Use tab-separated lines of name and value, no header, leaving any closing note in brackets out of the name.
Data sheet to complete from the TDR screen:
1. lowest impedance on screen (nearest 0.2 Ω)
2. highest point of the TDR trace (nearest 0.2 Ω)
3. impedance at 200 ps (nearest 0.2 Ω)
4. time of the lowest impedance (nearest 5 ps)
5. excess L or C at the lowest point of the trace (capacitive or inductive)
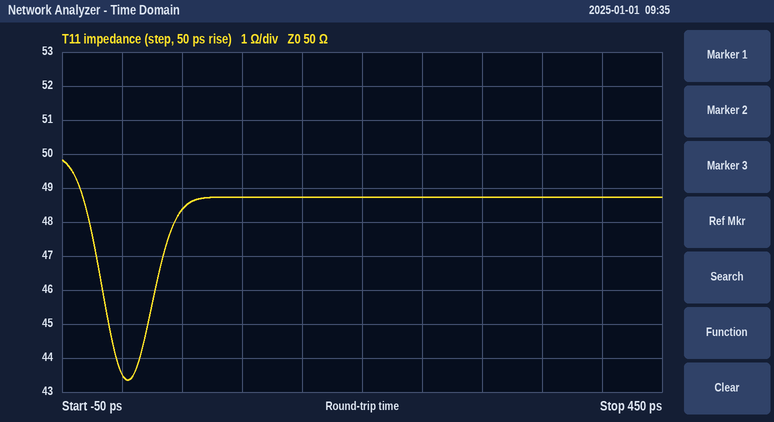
lowest impedance on screen	43.4 Ω
highest point of the TDR trace	49.8 Ω
impedance at 200 ps	48.8 Ω
time of the lowest impedance	5 ps
excess L or C at the lowest point of the trace	capacitive
